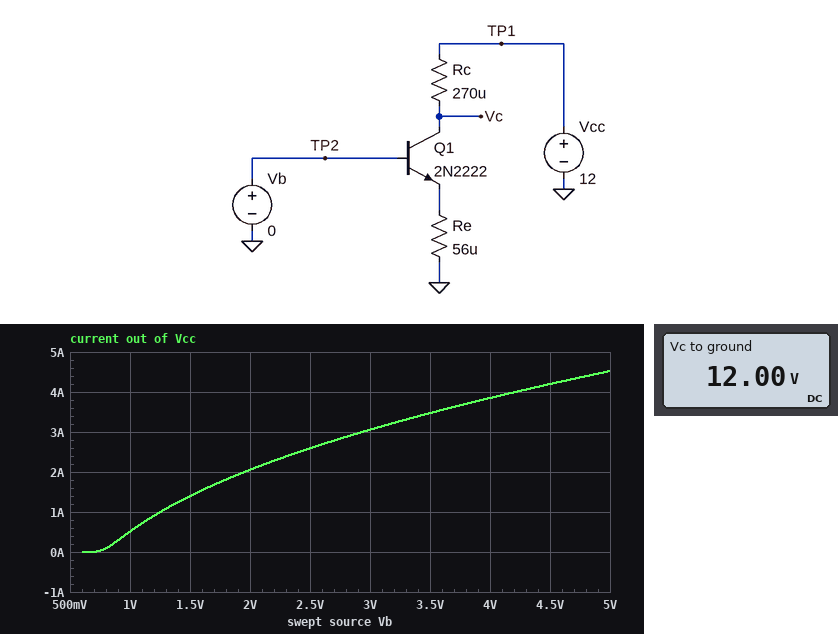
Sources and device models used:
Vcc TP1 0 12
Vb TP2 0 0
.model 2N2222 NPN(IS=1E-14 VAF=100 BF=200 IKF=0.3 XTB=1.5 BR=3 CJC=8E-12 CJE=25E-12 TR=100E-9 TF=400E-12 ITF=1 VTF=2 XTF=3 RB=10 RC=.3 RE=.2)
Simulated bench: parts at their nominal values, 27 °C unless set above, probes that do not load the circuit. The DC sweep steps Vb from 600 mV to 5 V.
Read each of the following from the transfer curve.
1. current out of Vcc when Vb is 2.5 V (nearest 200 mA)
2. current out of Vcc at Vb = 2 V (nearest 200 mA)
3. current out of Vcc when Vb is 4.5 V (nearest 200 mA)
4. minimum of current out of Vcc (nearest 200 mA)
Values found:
2.6 A
2.0 A
4.2 A
0 A
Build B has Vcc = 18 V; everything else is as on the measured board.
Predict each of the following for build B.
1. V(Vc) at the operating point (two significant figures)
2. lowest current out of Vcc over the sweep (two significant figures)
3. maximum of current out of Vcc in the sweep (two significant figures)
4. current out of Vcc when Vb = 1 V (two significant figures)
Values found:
18 V
140 µA
4.7 A
530 mA
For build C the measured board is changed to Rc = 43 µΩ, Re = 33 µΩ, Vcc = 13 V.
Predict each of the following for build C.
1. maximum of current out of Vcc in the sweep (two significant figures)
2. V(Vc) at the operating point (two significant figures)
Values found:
4.6 A
13 V
